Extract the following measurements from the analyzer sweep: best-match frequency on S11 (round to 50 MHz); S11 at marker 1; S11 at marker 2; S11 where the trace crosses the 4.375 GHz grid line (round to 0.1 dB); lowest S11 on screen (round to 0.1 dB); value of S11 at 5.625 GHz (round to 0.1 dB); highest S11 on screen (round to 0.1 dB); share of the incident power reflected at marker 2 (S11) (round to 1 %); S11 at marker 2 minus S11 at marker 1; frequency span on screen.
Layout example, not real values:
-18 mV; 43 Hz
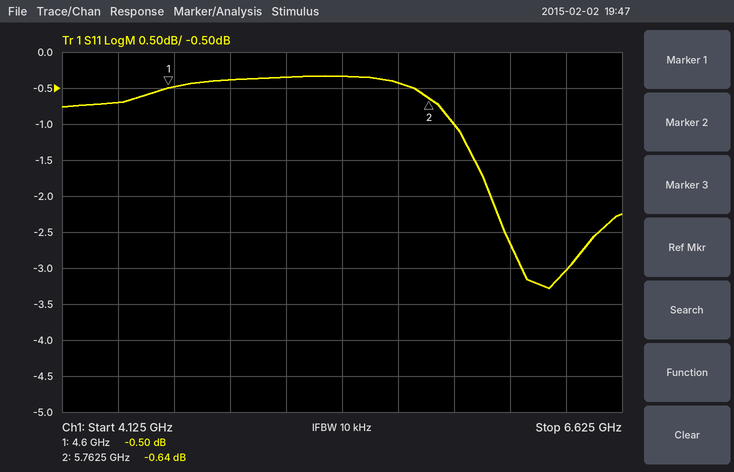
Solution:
6.30 GHz; -0.50 dB; -0.64 dB; -0.7 dB; -3.3 dB; -0.4 dB; -0.3 dB; 86 %; -0.14 dB; 2.5 GHz
